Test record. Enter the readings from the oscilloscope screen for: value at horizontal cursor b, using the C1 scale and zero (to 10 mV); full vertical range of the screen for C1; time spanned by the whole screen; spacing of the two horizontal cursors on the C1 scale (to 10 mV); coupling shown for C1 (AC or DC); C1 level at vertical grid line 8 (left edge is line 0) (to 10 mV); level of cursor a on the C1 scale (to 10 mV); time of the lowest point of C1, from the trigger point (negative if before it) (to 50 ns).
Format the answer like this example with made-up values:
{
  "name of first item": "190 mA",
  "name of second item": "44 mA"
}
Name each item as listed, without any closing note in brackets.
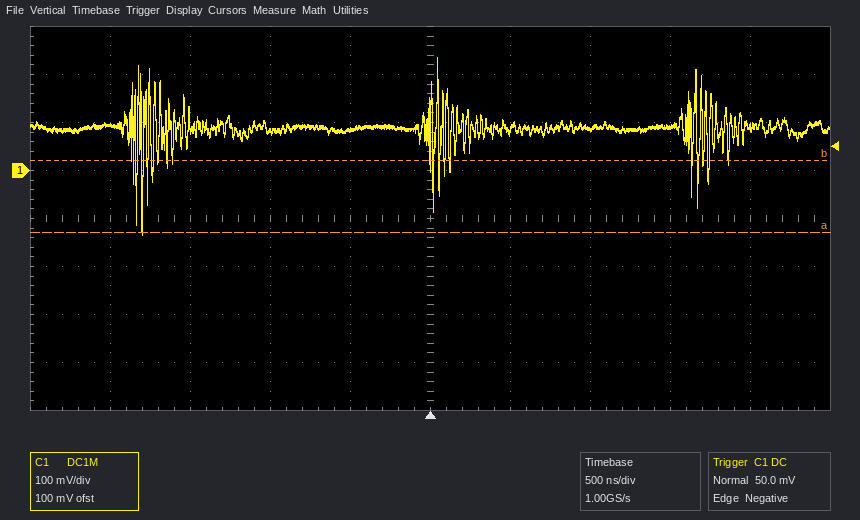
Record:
{
  "value at horizontal cursor b, using the C1 scale and zero": "20 mV",
  "full vertical range of the screen for C1": "800 mV",
  "time spanned by the whole screen": "5 µs",
  "spacing of the two horizontal cursors on the C1 scale": "150 mV",
  "coupling shown for C1": "DC",
  "C1 level at vertical grid line 8 (left edge is line 0)": "90 mV",
  "level of cursor a on the C1 scale": "-130 mV",
  "time of the lowest point of C1, from the trigger point (negative if before it)": "-1.80 µs"
}
